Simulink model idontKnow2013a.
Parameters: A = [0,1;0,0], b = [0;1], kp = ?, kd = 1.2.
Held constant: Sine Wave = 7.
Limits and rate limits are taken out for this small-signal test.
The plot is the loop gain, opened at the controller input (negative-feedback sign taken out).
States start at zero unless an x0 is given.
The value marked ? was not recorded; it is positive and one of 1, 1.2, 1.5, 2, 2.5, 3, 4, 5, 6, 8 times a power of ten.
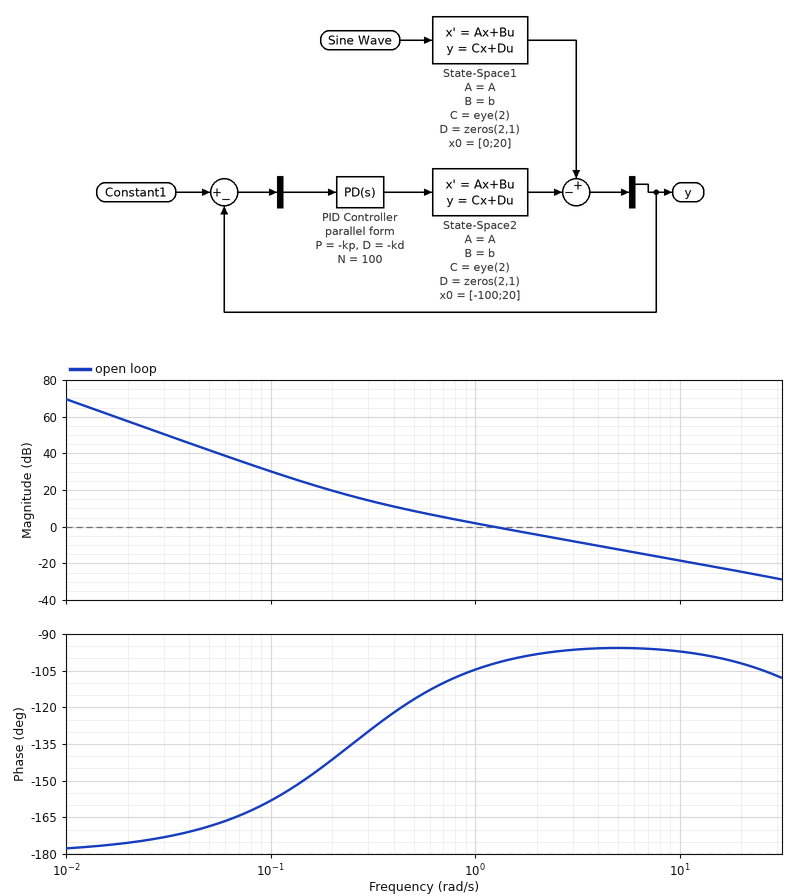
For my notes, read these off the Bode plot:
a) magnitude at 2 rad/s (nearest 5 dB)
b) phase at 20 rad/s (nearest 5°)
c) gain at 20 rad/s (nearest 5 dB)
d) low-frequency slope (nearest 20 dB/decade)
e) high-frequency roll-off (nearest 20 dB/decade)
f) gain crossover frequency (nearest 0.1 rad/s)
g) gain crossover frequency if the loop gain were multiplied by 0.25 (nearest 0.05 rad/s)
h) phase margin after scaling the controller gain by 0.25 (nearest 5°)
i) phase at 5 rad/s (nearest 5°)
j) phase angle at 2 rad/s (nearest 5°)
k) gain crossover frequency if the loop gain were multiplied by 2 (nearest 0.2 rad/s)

-5 dB
-100°
-25 dB
-40 dB/decade
-20 dB/decade
1.2 rad/s
0.35 rad/s
55°
-95°
-100°
2.4 rad/s
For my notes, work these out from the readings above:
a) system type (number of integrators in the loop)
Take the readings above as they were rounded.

2
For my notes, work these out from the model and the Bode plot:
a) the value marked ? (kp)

0.3
